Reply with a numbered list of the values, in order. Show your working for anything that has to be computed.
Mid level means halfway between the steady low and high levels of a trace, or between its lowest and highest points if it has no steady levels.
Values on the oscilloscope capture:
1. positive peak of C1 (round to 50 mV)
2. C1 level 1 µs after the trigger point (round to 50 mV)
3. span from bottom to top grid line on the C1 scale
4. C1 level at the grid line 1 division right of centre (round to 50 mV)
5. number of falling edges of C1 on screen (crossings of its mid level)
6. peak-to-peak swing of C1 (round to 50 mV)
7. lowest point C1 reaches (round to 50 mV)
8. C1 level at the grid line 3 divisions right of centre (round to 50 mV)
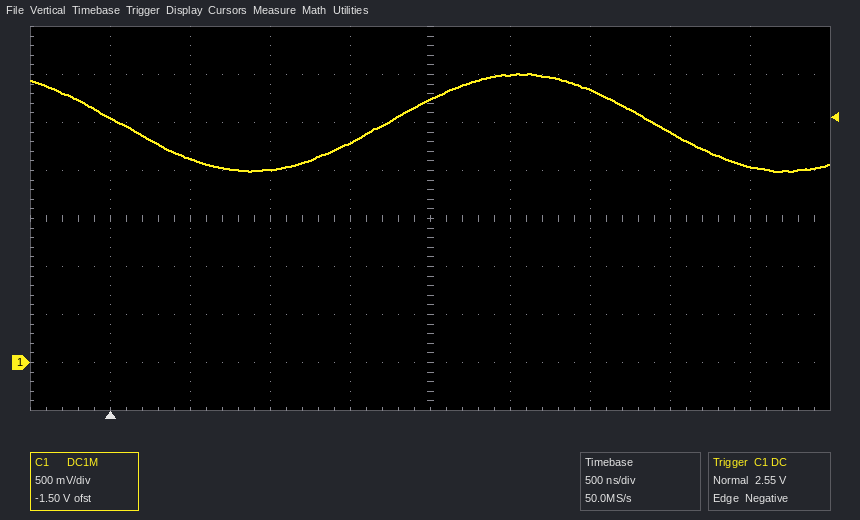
1. 3.00 V
2. 2.00 V
3. 4 V
4. 3.00 V
5. 2
6. 3.00 V − (2.00 V) = 1.00 V
7. 2.00 V
8. 2.40 V
